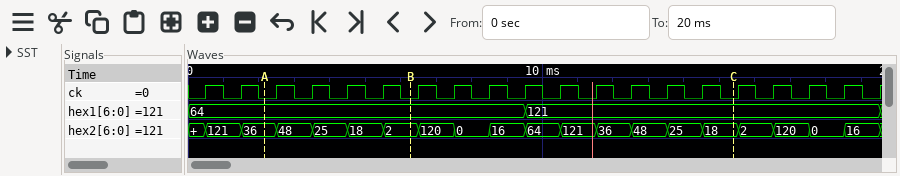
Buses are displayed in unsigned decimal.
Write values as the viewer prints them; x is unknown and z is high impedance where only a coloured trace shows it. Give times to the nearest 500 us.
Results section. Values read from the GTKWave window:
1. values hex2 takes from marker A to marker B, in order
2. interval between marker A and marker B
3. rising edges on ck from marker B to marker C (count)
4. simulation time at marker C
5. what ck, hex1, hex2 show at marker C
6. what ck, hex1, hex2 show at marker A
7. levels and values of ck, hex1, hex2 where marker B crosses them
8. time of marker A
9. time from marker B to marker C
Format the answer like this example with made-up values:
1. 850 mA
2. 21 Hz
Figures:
1. 36, 48, 25, 18, 2
2. 4000 us
3. 9
4. 15500 us
5. ck=0, hex1=121, hex2=18
6. ck=0, hex1=64, hex2=36
7. ck=0, hex1=64, hex2=2
8. 2000 us
9. 9000 us
